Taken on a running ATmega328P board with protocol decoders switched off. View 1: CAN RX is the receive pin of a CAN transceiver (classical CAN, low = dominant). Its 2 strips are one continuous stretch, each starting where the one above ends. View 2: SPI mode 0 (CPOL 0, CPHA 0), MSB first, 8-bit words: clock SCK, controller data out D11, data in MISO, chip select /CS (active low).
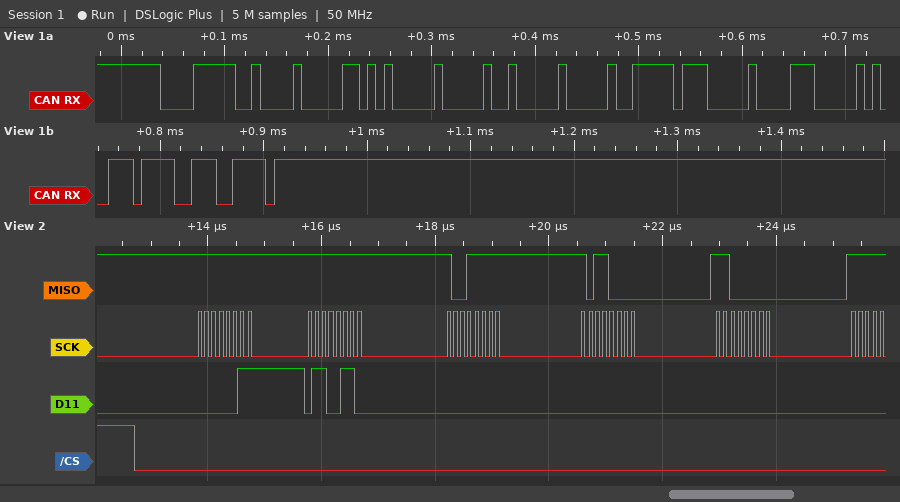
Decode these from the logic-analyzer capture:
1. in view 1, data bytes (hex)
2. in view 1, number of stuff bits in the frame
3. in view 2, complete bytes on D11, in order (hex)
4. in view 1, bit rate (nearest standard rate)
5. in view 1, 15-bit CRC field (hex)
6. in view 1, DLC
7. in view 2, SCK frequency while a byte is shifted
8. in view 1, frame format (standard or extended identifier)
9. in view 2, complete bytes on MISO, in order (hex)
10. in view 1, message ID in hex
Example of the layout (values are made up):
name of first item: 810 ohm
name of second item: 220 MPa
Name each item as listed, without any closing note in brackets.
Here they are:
in view 1, data bytes: 2A 00 10 00 FF 00 70 27
in view 1, number of stuff bits in the frame: 9
in view 2, complete bytes on D11, in order: 03 66 00 00 00
in view 1, bit rate: 125 kbit/s
in view 1, 15-bit CRC field: 0x3CE7
in view 1, DLC: 8
in view 2, SCK frequency while a byte is shifted: 8 MHz
in view 1, frame format: standard
in view 2, complete bytes on MISO, in order: FF FF 9F B0 C0
in view 1, message ID in hex: 0x0FA
